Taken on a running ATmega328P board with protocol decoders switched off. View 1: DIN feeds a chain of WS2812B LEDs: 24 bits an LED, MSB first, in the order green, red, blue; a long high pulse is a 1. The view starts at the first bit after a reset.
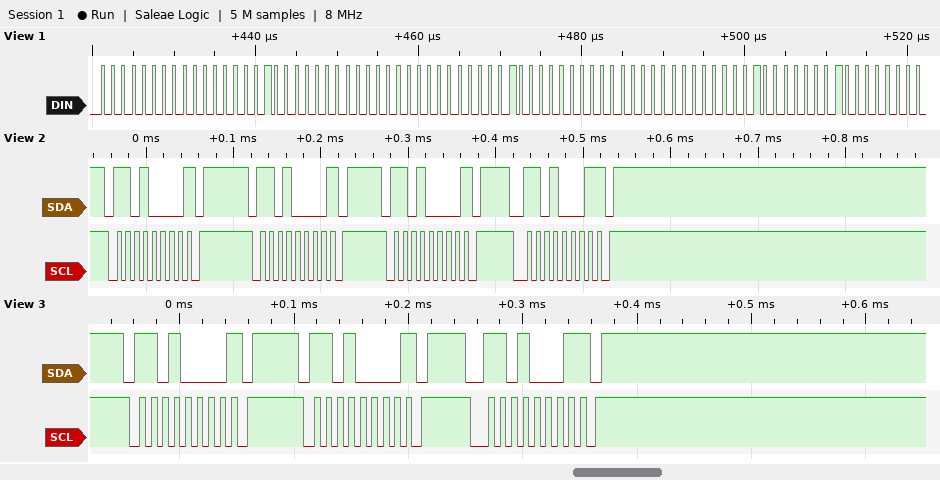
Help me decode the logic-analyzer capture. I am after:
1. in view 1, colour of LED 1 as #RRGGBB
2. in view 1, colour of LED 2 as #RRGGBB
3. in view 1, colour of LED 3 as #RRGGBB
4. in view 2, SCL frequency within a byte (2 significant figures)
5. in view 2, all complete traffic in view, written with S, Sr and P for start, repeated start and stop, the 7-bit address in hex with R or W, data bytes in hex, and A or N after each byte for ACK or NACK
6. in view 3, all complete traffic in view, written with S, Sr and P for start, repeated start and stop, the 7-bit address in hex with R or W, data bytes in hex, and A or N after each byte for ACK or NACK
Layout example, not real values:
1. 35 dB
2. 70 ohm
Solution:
1. #000080
2. #000080
3. #000080
4. 100 kHz
5. S 68W N P S 68W N P S 68W N P S 68R N P
6. S 68W N P S 68W N P S 68R N P
